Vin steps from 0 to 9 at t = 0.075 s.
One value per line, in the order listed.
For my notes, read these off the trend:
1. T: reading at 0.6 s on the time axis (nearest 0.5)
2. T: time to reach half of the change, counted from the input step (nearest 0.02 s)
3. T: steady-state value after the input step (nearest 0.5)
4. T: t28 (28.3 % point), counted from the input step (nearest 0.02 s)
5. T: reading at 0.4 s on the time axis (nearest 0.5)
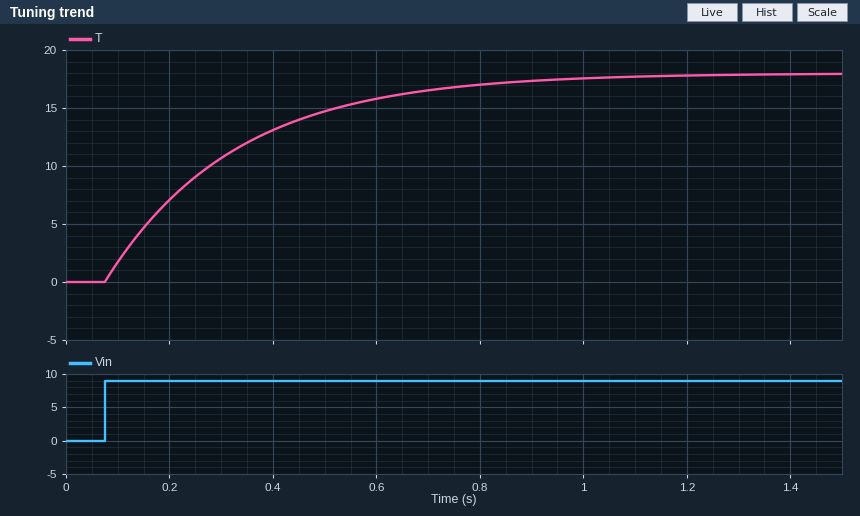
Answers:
16.0
0.18 s
18.0
0.08 s
13.0
